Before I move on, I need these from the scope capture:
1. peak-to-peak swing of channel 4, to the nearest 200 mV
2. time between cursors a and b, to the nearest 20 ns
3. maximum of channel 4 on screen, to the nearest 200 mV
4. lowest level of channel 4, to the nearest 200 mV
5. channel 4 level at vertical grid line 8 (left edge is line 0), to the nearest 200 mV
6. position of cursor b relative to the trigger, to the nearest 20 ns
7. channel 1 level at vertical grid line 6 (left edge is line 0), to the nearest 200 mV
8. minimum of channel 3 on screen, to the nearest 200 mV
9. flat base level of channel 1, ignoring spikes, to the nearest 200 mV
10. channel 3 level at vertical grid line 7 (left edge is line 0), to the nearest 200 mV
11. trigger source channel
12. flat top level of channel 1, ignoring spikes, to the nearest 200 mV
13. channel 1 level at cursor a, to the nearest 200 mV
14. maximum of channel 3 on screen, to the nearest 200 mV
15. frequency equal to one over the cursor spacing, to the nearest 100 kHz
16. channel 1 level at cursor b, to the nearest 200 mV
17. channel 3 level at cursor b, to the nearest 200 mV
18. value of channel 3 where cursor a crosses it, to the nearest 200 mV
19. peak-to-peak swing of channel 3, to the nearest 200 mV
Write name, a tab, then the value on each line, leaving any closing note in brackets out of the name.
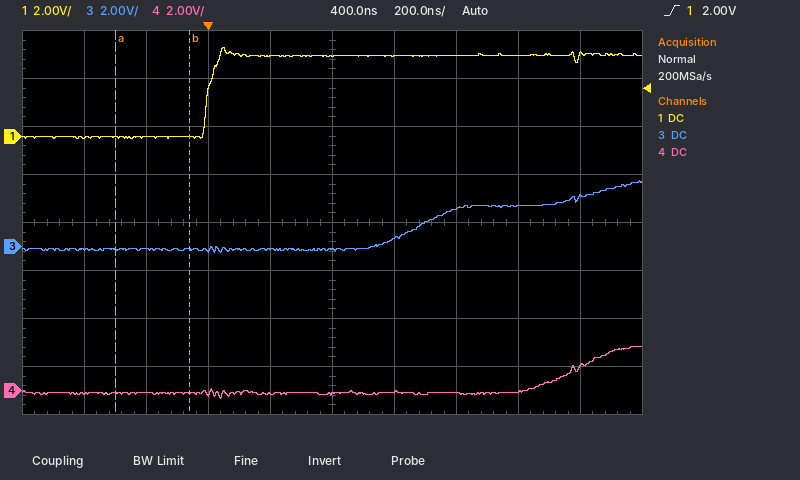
peak-to-peak swing of channel 4, to the nearest 200 mV	2.2 V
time between cursors a and b, to the nearest 20 ns	240 ns
maximum of channel 4 on screen, to the nearest 200 mV	1.8 V
lowest level of channel 4, to the nearest 200 mV	-400 mV
channel 4 level at vertical grid line 8 (left edge is line 0), to the nearest 200 mV	0.0 V
position of cursor b relative to the trigger, to the nearest 20 ns	-60 ns
channel 1 level at vertical grid line 6 (left edge is line 0), to the nearest 200 mV	3.4 V
minimum of channel 3 on screen, to the nearest 200 mV	-200 mV
flat base level of channel 1, ignoring spikes, to the nearest 200 mV	0.0 V
channel 3 level at vertical grid line 7 (left edge is line 0), to the nearest 200 mV	1.6 V
trigger source channel	channel 1
flat top level of channel 1, ignoring spikes, to the nearest 200 mV	3.4 V
channel 1 level at cursor a, to the nearest 200 mV	0.0 V
maximum of channel 3 on screen, to the nearest 200 mV	2.8 V
frequency equal to one over the cursor spacing, to the nearest 100 kHz	4.2 MHz
channel 1 level at cursor b, to the nearest 200 mV	0.0 V
channel 3 level at cursor b, to the nearest 200 mV	-200 mV
value of channel 3 where cursor a crosses it, to the nearest 200 mV	-200 mV
peak-to-peak swing of channel 3, to the nearest 200 mV	3.0 V
